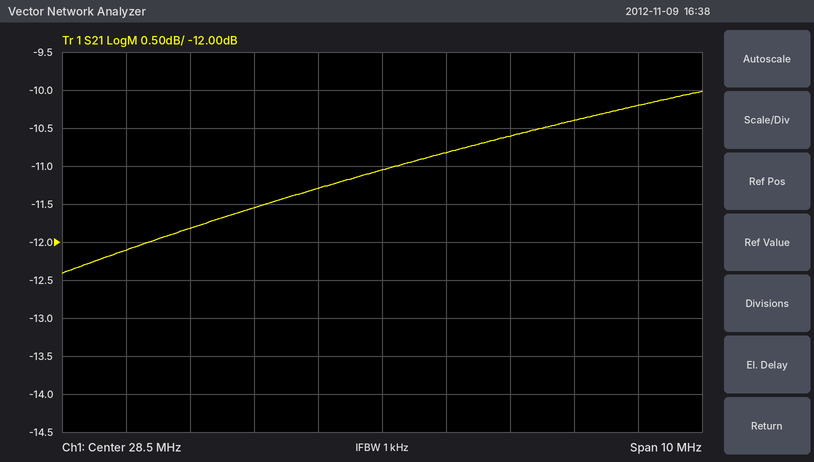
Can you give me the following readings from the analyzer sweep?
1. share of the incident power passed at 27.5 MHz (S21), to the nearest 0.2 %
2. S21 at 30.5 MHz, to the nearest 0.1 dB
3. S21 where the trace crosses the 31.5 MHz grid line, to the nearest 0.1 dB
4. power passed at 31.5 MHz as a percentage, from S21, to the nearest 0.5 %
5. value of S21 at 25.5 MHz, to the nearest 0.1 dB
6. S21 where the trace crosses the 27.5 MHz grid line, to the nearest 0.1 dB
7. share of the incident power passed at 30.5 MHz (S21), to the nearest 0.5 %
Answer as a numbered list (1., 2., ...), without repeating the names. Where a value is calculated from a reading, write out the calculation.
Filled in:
1. 10^(-11.3/10) ≈ 7.4 %
2. -10.6 dB
3. -10.4 dB
4. 10^(-10.4/10) ≈ 9.12 %, so 9.0 % to the nearest 0.5 %
5. -11.8 dB
6. -11.3 dB
7. 10^(-10.6/10) ≈ 8.71 %, so 8.5 % to the nearest 0.5 %
